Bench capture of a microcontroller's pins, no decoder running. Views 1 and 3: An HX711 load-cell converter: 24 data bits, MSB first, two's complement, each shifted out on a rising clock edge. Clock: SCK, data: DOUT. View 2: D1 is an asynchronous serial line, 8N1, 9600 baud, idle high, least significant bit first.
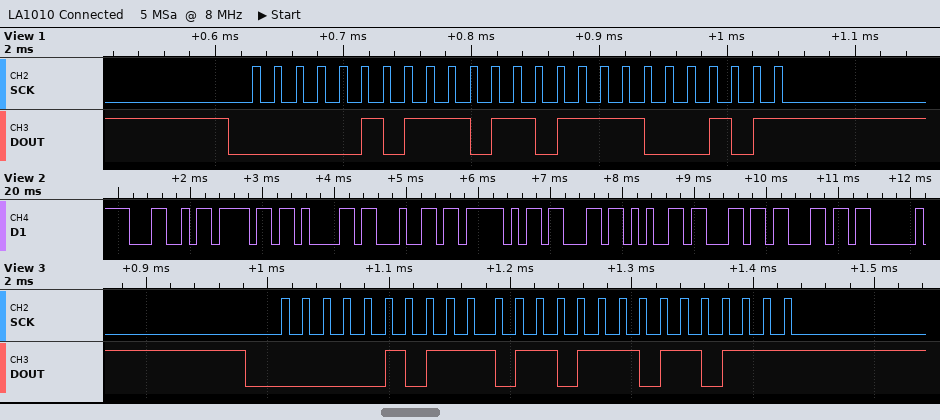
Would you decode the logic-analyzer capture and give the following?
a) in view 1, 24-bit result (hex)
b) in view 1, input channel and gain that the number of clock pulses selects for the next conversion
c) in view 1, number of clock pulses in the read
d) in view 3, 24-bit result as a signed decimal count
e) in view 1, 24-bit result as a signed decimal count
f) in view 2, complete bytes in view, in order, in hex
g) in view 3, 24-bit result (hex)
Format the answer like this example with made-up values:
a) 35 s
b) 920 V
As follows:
a) 0x05DBC5
b) channel A, gain 128
c) 25
d) 383927
e) 383941
f) 4C 6F 61 64 5F 63 65 6C 6C
g) 0x05DBB7
